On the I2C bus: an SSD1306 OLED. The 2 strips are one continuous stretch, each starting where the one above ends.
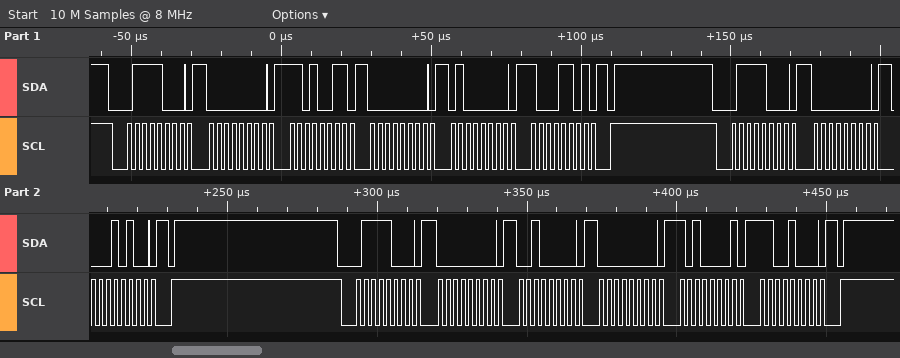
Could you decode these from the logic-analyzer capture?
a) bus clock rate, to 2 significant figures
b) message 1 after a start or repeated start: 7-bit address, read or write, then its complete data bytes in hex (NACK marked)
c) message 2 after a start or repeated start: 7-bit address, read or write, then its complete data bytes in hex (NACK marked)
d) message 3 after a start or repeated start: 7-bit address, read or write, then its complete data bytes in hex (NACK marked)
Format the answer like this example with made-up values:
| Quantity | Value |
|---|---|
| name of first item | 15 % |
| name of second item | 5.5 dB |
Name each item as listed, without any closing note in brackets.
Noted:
| Quantity | Value |
|---|---|
| bus clock rate, to 2 significant figures | 400 kHz |
| message 1 after a start or repeated start: 7-bit address, read or write, then its complete data bytes in hex | 0x3C write: 00 D3 00 40 8D |
| message 2 after a start or repeated start: 7-bit address, read or write, then its complete data bytes in hex | 0x3C write: 00 14 |
| message 3 after a start or repeated start: 7-bit address, read or write, then its complete data bytes in hex | 0x3C write: 00 20 00 A1 C8 |
